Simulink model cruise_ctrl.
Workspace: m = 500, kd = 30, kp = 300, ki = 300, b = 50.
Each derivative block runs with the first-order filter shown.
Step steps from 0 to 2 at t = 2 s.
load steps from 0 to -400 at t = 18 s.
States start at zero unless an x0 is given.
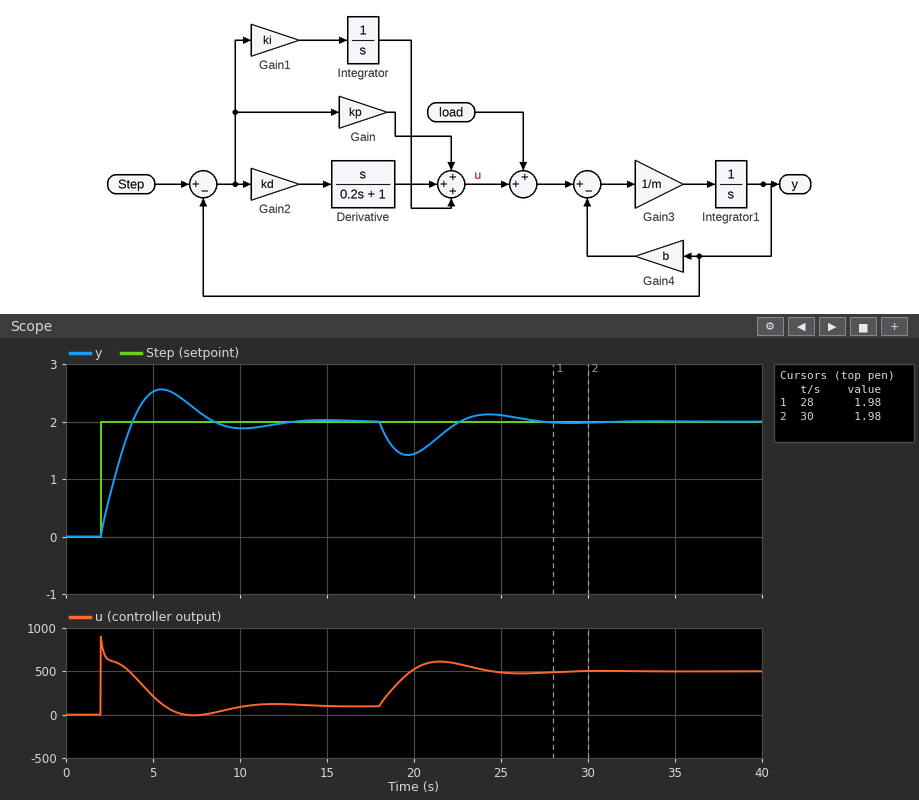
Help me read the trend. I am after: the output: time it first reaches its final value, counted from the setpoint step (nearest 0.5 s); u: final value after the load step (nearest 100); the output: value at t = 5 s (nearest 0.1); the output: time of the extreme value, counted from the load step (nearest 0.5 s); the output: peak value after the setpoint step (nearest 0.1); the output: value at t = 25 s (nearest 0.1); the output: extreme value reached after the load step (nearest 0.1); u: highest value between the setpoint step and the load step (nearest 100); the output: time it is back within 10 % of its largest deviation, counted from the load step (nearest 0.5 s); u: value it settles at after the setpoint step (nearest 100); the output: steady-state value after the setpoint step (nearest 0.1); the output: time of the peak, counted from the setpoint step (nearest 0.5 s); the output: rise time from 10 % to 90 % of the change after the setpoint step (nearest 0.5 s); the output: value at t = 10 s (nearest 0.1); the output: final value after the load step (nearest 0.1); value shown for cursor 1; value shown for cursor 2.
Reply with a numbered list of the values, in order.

1. 2.0 s
2. 500
3. 2.5
4. 1.5 s
5. 2.6
6. 2.1
7. 1.4
8. 900
9. 8.0 s
10. 100
11. 2.0
12. 3.5 s
13. 1.5 s
14. 1.9
15. 2.0
16. 1.98
17. 1.98
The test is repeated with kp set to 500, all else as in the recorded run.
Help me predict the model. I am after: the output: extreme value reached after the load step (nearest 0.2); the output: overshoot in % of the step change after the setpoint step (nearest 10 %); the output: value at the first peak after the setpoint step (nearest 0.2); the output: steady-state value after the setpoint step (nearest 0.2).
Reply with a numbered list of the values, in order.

1. 1.6
2. 20 %
3. 2.4
4. 2.0
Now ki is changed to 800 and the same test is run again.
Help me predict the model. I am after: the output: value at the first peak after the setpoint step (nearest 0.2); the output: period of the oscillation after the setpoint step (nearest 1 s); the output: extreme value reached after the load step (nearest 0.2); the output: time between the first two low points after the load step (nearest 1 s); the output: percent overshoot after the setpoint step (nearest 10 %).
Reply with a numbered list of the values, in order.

1. 2.8
2. 5 s
3. 1.6
4. 5 s
5. 40 %
